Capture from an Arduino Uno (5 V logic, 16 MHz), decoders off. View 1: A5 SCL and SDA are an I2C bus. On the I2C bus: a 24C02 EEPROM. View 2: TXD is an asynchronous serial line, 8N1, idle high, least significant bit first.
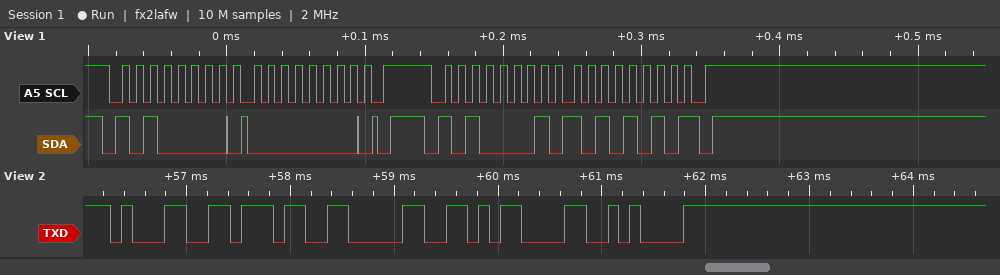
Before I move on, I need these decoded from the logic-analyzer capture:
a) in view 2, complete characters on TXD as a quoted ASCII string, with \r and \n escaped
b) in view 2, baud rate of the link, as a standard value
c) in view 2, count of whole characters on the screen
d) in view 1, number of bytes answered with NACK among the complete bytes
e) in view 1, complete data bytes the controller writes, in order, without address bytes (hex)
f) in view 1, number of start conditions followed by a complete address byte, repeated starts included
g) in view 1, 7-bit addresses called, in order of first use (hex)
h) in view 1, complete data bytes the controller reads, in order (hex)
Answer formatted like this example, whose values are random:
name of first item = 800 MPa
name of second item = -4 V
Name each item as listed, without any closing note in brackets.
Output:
in view 2, complete characters on TXD as a quoted ASCII string, with \r and \n escaped = "170\r\n"
in view 2, baud rate of the link, as a standard value = 9600 baud
in view 2, count of whole characters on the screen = 5
in view 1, number of bytes answered with NACK among the complete bytes = 1
in view 1, complete data bytes the controller writes, in order, without address bytes = 00
in view 1, number of start conditions followed by a complete address byte, repeated starts included = 2
in view 1, 7-bit addresses called, in order of first use = 0x50
in view 1, complete data bytes the controller reads, in order = AA
